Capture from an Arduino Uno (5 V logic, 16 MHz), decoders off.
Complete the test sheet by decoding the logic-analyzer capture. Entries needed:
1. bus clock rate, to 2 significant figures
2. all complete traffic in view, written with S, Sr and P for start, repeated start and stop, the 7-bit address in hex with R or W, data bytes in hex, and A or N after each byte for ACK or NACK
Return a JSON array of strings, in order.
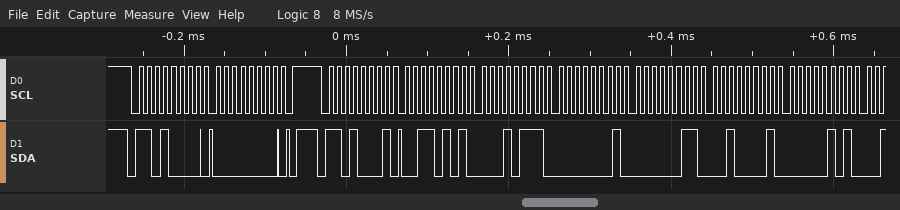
["100 kHz", "S 68W A 00 A P S 68R A 35 A 17 A 01 A 03 A 21 A 05 A"]
